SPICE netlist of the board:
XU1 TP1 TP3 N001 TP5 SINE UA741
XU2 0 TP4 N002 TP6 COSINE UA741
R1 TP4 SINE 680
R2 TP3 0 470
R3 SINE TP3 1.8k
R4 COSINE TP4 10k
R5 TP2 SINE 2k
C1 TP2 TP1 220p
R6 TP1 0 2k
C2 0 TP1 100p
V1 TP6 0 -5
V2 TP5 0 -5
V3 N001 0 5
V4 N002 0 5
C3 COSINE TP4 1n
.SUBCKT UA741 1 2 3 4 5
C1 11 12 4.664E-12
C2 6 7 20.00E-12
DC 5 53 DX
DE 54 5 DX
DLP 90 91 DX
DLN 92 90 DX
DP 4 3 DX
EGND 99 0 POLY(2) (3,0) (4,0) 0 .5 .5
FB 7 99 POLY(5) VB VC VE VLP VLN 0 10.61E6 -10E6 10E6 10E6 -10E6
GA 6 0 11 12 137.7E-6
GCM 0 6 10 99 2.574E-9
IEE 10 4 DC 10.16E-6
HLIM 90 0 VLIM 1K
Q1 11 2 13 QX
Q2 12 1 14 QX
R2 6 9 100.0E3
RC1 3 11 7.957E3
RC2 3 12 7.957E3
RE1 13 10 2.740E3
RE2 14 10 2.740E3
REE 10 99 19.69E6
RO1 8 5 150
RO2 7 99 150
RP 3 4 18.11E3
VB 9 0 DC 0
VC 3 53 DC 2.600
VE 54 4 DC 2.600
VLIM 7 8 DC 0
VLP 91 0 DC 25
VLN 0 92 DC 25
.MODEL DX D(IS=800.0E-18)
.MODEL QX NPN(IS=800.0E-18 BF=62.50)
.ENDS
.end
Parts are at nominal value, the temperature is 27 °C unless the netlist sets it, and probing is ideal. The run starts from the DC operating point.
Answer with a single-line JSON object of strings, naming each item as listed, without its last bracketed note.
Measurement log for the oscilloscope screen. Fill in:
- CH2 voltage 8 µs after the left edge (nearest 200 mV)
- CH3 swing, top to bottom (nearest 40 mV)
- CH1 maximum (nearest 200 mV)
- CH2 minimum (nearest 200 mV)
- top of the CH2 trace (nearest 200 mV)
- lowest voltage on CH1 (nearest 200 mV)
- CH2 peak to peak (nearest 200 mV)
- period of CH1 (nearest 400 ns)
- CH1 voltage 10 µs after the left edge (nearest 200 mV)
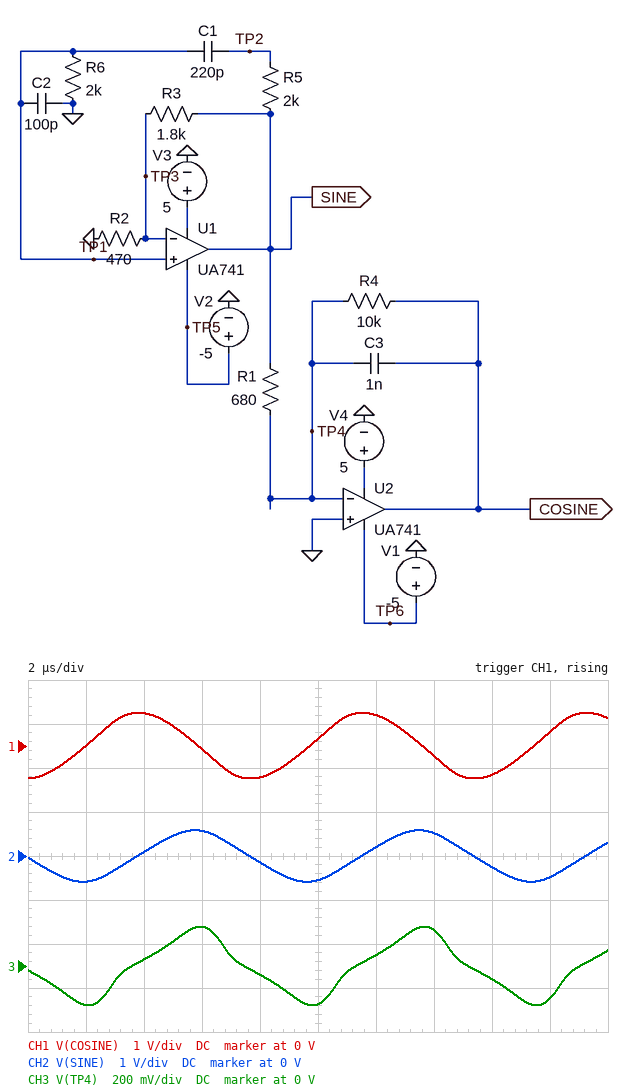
{"CH2 voltage 8 µs after the left edge": "-200 mV", "CH3 swing, top to bottom": "360 mV", "CH1 maximum": "800 mV", "CH2 minimum": "-600 mV", "top of the CH2 trace": "600 mV", "lowest voltage on CH1": "-800 mV", "CH2 peak to peak": "1.2 V", "period of CH1": "7.6 µs", "CH1 voltage 10 µs after the left edge": "200 mV"}
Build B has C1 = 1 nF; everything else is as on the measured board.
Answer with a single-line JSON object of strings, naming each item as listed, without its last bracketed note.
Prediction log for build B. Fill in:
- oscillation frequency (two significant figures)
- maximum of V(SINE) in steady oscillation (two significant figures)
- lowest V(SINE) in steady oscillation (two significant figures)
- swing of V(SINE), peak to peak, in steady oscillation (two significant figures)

{"oscillation frequency": "33 kHz", "maximum of V(SINE) in steady oscillation": "3.0 V", "lowest V(SINE) in steady oscillation": "-3.0 V", "swing of V(SINE), peak to peak, in steady oscillation": "6.0 V"}
